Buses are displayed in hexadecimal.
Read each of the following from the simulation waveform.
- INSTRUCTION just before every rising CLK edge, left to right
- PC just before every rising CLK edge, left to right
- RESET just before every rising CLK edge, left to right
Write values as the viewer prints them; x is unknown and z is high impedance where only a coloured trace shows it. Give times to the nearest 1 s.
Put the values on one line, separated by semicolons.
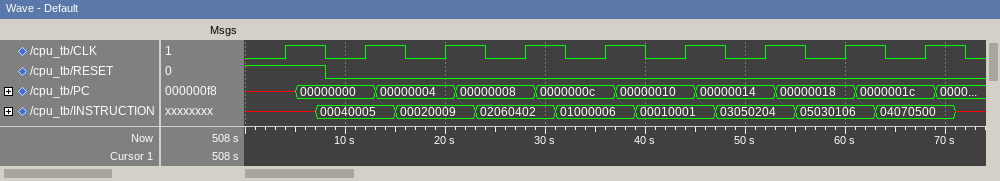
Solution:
x, 00040005, 00020009, 02060402, 01000006, 00010001, 03050204, 05030106, 04070500; x, 00000000, 00000004, 00000008, 0000000c, 00000010, 00000014, 00000018, 0000001c; 1 0 0 0 0 0 0 0 0
